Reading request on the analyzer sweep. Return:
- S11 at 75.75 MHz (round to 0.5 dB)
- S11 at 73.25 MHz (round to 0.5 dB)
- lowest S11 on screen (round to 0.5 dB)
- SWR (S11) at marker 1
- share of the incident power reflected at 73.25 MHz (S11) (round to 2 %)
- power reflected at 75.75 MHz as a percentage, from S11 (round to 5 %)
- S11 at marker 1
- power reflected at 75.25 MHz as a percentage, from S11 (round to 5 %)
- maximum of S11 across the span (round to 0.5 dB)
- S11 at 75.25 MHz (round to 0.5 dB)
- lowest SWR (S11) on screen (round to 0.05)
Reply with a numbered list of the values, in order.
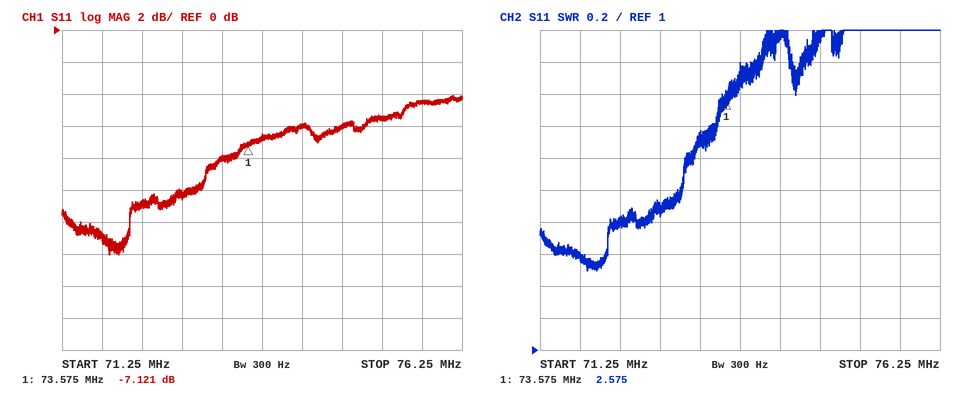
1. -4.5 dB
2. -8.0 dB
3. -14.0 dB
4. 2.575
5. 16 %
6. 35 %
7. -7.121 dB
8. 30 %
9. -4.0 dB
10. -5.5 dB
11. 1.50
